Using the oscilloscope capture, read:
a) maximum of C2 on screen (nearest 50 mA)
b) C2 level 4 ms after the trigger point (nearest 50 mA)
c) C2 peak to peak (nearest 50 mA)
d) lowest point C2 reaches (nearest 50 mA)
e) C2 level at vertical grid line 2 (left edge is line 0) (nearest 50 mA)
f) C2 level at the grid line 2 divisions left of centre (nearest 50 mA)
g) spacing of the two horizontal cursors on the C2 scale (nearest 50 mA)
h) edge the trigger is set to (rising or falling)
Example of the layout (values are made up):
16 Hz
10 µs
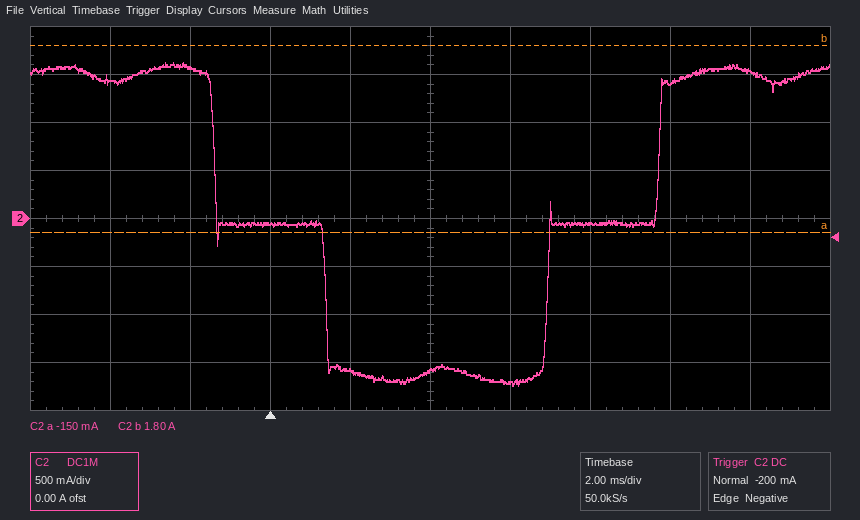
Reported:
1.60 A
-1.60 A
3.35 A
-1.75 A
1.55 A
-50 mA
1.95 A
falling
